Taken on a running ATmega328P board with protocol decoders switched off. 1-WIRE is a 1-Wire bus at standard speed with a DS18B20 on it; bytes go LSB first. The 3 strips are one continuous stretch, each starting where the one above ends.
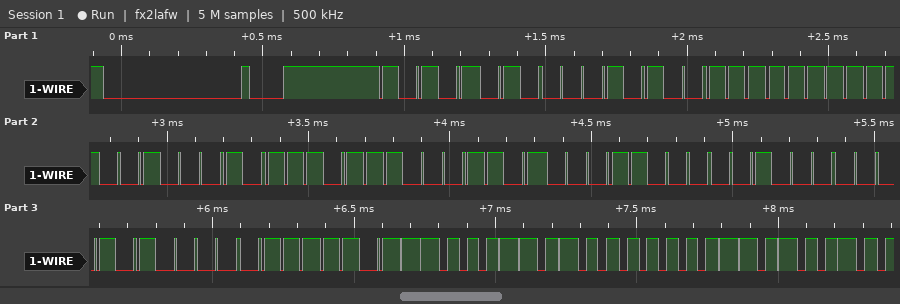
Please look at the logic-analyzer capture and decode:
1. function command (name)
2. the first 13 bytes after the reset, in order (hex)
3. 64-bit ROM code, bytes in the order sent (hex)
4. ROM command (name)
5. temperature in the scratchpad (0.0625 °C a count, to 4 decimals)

Read Scratchpad
55 28 FF 13 DD B1 18 04 0A BE 63 01 4B
28 FF 13 DD B1 18 04 0A
Match ROM
22.1875 °C
